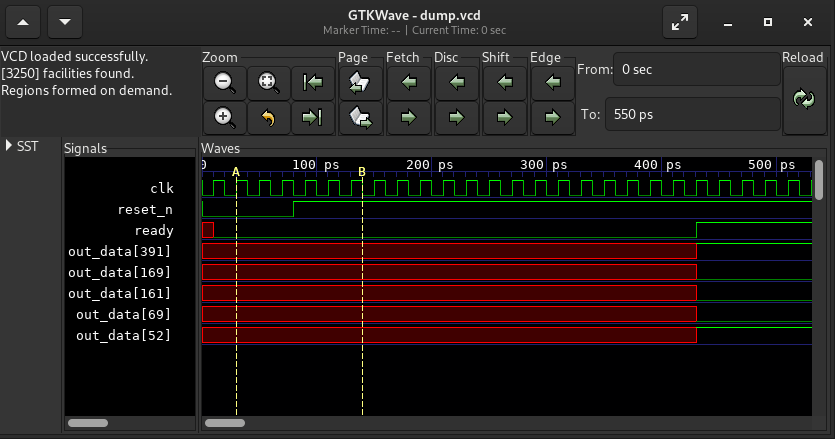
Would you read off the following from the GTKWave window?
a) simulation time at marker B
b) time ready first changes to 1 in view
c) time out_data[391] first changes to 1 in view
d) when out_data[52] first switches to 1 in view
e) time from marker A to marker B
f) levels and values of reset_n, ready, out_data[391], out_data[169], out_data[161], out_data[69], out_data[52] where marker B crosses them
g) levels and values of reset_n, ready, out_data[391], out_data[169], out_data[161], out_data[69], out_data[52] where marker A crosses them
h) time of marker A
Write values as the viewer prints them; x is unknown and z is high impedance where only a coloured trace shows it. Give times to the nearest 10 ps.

140 ps
430 ps
430 ps
430 ps
110 ps
reset_n=1, ready=0, out_data[391]=x, out_data[169]=x, out_data[161]=x, out_data[69]=x, out_data[52]=x
reset_n=0, ready=0, out_data[391]=x, out_data[169]=x, out_data[161]=x, out_data[69]=x, out_data[52]=x
30 ps
